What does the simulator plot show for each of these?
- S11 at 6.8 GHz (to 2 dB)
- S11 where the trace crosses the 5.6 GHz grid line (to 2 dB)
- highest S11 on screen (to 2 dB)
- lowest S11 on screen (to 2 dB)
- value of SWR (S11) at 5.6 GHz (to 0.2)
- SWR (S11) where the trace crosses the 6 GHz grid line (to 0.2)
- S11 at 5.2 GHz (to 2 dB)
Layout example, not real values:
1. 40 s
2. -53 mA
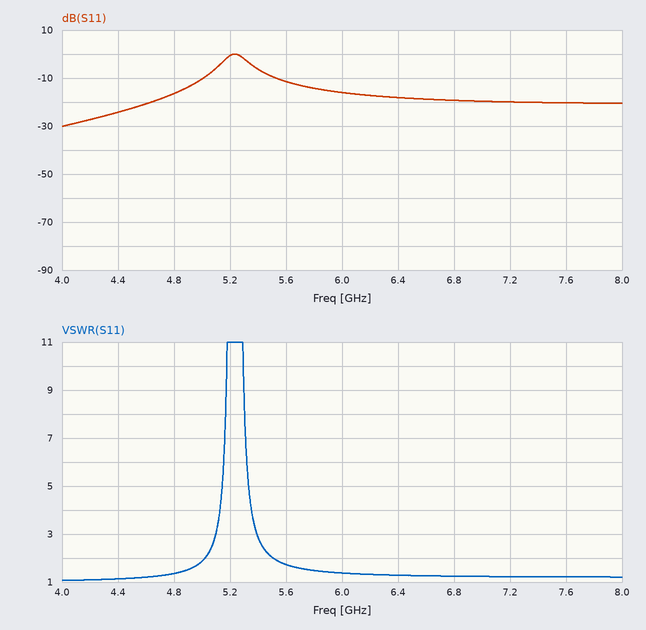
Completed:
1. -20 dB
2. -12 dB
3. 0 dB
4. -30 dB
5. 1.8
6. 1.4
7. 0 dB
